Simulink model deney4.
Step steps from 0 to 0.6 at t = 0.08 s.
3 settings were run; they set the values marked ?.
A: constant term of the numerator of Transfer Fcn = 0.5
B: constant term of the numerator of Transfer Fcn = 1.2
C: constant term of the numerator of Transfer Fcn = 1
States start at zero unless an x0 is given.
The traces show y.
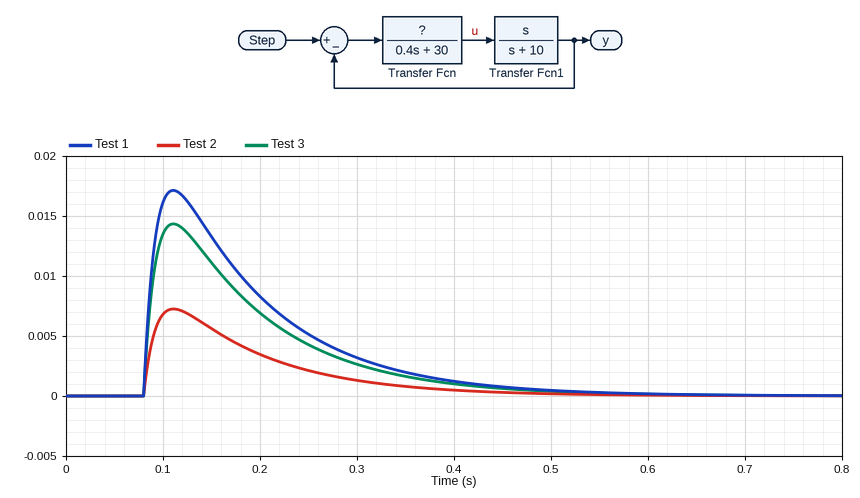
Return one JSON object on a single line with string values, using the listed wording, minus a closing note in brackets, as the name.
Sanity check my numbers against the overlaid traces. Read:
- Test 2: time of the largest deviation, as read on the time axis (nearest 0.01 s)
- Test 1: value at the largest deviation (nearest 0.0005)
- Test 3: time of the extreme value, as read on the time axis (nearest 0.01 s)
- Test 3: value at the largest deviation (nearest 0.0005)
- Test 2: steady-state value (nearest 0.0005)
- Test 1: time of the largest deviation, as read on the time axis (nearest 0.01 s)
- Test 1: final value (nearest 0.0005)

{"Test 2: time of the largest deviation, as read on the time axis": "0.11 s", "Test 1: value at the largest deviation": "0.0170", "Test 3: time of the extreme value, as read on the time axis": "0.11 s", "Test 3: value at the largest deviation": "0.0145", "Test 2: steady-state value": "0.0000", "Test 1: time of the largest deviation, as read on the time axis": "0.11 s", "Test 1: final value": "0.0000"}
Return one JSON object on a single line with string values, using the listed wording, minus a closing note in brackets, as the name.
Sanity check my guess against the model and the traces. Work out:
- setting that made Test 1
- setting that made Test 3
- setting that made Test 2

{"setting that made Test 1": "B", "setting that made Test 3": "C", "setting that made Test 2": "A"}
